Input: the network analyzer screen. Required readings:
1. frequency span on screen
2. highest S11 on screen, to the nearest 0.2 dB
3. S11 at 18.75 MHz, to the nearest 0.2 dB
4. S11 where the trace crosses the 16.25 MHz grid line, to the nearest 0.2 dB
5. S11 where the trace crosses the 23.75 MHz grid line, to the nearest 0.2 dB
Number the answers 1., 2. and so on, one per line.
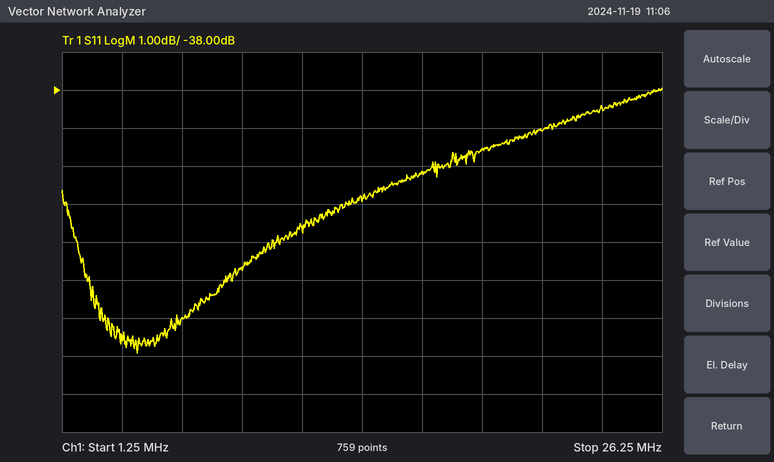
1. 25 MHz
2. -38.0 dB
3. -39.6 dB
4. -40.2 dB
5. -38.4 dB
